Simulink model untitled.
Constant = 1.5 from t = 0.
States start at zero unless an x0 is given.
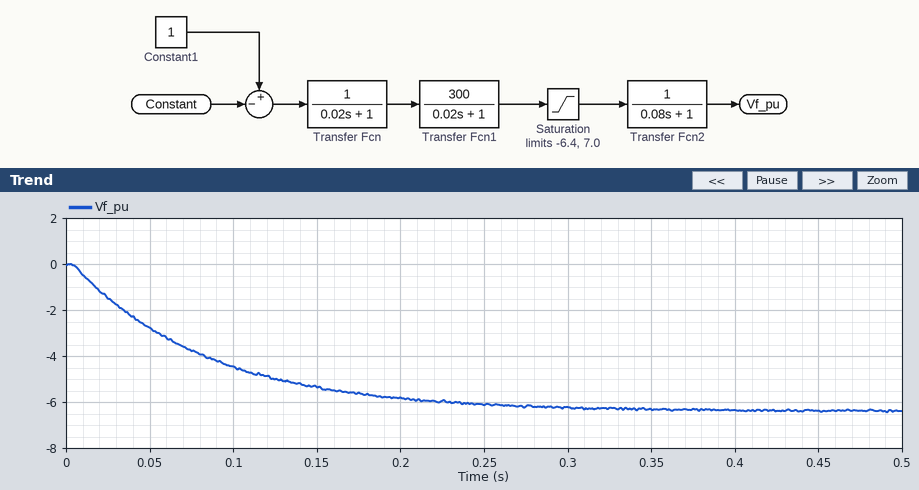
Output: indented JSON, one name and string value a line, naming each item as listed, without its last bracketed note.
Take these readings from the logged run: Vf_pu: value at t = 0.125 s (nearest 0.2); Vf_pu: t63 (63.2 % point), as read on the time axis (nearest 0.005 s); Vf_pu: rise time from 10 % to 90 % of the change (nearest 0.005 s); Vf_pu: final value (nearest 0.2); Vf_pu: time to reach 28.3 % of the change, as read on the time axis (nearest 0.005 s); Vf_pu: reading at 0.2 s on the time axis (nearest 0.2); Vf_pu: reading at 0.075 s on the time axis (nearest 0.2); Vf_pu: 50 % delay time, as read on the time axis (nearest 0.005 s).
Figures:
{
  "Vf_pu: value at t = 0.125 s": "-5.0",
  "Vf_pu: t63 (63.2 % point), as read on the time axis": "0.085 s",
  "Vf_pu: rise time from 10 % to 90 % of the change": "0.175 s",
  "Vf_pu: final value": "-6.4",
  "Vf_pu: time to reach 28.3 % of the change, as read on the time axis": "0.030 s",
  "Vf_pu: reading at 0.2 s on the time axis": "-5.8",
  "Vf_pu: reading at 0.075 s on the time axis": "-3.8",
  "Vf_pu: 50 % delay time, as read on the time axis": "0.060 s"
}
